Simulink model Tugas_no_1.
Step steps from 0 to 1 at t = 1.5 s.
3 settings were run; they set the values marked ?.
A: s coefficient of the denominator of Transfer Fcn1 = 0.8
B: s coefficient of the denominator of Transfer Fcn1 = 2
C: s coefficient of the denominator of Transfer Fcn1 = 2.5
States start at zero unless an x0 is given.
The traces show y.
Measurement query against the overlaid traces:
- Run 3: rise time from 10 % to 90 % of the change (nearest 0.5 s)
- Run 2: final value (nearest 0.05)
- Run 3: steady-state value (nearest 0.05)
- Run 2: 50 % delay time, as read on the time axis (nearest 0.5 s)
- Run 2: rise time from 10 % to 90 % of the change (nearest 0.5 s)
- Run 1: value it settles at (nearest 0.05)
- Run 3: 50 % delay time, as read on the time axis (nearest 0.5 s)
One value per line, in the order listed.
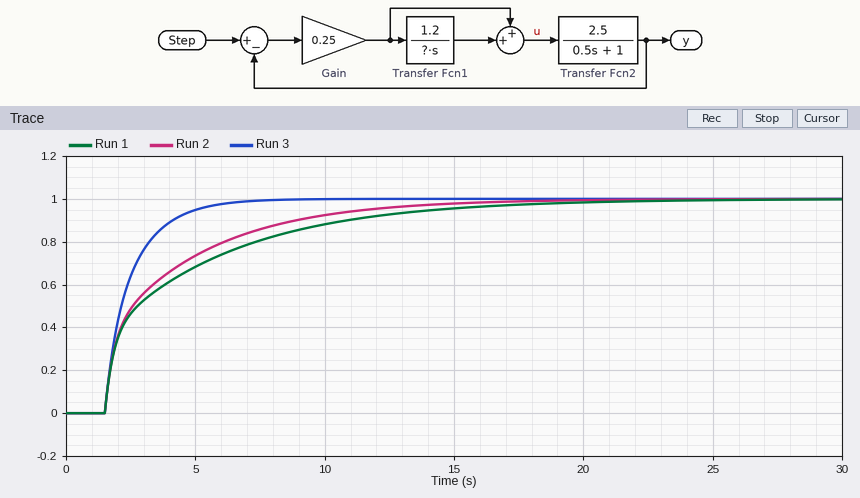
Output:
2.5 s
1.00
1.00
2.5 s
7.5 s
1.00
2.0 s
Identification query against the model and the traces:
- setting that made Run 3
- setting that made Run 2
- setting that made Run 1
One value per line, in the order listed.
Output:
A
B
C
